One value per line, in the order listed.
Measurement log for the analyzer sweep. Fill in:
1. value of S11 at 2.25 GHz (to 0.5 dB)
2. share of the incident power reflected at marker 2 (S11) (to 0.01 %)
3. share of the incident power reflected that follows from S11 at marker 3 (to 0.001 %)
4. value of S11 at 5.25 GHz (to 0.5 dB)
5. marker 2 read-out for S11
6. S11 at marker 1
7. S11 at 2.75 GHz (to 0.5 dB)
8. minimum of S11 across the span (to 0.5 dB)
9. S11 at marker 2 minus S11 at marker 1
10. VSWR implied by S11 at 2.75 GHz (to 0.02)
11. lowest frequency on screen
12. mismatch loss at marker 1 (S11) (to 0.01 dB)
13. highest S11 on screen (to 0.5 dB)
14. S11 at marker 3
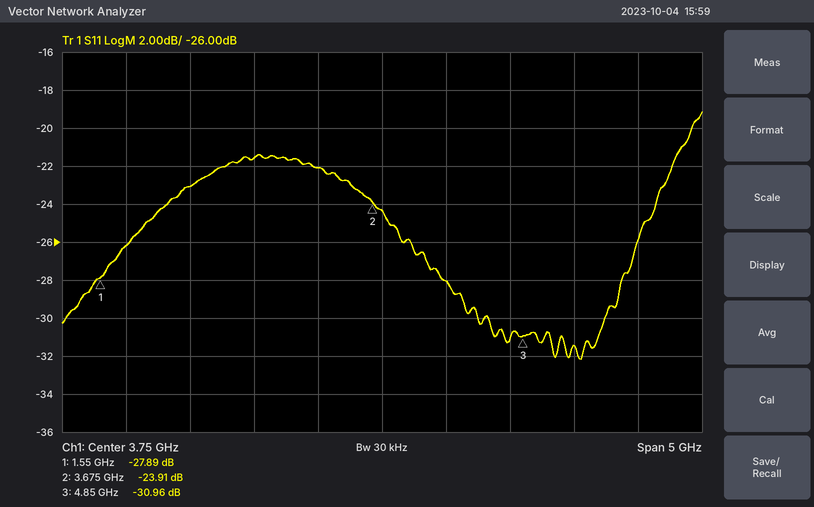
-23.0 dB
0.41 %
0.080 %
-31.5 dB
-23.91 dB
-27.89 dB
-21.5 dB
-32.0 dB
3.98 dB
1.18
1.25 GHz
0.01 dB
-19.0 dB
-30.96 dB
